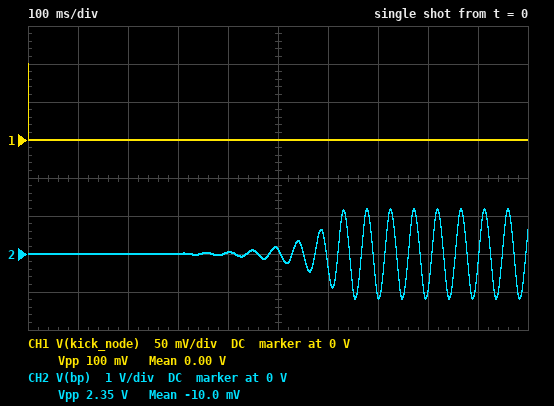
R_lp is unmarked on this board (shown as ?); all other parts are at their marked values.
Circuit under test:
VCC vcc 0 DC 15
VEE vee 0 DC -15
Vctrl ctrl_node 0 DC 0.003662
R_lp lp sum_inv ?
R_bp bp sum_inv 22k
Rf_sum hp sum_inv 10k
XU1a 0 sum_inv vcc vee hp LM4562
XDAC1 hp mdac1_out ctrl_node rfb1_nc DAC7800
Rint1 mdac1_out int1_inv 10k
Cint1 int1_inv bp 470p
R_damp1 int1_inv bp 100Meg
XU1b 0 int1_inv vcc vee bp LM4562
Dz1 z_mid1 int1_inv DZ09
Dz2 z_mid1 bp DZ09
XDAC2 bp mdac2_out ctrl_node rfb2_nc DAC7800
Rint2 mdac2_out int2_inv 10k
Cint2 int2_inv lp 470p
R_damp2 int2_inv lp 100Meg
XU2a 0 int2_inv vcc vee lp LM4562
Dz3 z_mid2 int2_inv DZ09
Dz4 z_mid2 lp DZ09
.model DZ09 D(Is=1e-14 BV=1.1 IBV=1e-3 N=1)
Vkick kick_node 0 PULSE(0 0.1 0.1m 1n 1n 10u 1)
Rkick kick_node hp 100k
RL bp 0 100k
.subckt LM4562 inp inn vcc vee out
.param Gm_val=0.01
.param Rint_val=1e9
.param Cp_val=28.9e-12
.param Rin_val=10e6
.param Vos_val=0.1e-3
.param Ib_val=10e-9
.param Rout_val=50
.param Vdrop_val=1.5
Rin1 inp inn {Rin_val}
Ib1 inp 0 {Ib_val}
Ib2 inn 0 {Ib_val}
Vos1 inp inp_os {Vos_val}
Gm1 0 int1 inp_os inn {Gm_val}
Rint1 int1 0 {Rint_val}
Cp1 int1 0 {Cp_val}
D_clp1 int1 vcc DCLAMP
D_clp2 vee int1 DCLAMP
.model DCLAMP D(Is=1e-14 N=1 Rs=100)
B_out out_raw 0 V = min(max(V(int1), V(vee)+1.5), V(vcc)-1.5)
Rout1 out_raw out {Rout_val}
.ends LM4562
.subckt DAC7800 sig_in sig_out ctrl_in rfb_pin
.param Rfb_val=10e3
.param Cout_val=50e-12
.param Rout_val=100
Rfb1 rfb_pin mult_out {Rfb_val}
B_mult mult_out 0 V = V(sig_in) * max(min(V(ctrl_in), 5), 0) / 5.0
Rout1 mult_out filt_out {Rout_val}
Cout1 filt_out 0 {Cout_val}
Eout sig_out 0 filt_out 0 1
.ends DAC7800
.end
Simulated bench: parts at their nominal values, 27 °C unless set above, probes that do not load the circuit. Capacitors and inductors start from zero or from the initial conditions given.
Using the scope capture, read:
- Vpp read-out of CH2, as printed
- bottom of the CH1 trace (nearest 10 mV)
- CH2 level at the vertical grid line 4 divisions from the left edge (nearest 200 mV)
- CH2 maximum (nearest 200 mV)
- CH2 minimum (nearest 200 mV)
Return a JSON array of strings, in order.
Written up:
["2.35 V", "0 V", "0 V", "1.2 V", "-1.2 V"]
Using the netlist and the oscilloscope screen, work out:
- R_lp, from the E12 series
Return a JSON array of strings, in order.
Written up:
["12 kΩ"]
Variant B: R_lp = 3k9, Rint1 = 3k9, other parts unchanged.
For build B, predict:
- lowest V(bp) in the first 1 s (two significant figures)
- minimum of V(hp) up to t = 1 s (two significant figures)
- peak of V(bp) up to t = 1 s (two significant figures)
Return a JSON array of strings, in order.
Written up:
["-1.3 V", "-1.7 V", "1.3 V"]
